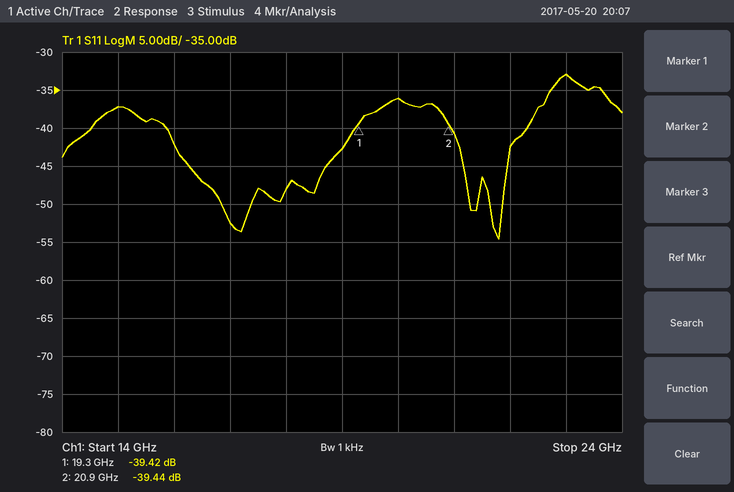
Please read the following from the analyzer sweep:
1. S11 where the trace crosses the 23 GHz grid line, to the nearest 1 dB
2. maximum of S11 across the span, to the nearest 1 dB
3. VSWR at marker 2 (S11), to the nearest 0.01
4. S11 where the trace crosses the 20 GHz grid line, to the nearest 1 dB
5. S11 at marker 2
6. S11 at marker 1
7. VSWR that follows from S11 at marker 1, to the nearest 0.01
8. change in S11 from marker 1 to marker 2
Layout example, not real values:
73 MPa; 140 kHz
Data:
-33 dB; -33 dB; 1.02; -36 dB; -39.44 dB; -39.42 dB; 1.02; -0.02 dB
